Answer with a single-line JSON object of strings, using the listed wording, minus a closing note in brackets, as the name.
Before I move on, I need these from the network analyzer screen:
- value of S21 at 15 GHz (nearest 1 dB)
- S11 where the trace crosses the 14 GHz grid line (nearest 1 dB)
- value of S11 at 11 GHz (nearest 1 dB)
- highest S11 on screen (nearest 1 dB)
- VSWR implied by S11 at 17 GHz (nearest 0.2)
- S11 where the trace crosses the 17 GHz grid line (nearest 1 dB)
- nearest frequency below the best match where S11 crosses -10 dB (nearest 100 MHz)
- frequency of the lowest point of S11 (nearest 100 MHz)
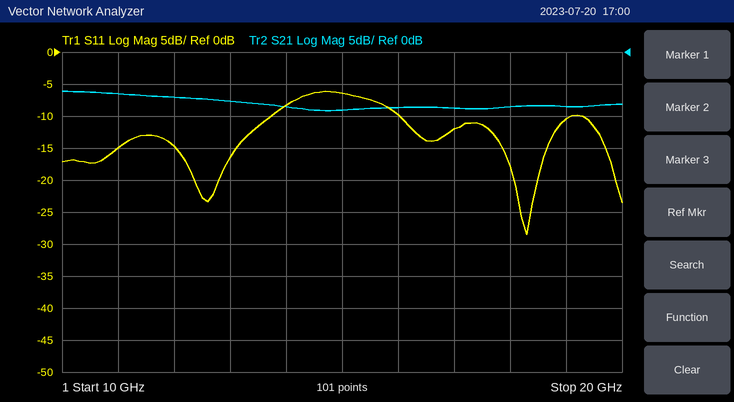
{"value of S21 at 15 GHz": "-9 dB", "S11 where the trace crosses the 14 GHz grid line": "-8 dB", "value of S11 at 11 GHz": "-15 dB", "highest S11 on screen": "-6 dB", "VSWR implied by S11 at 17 GHz": "1.6", "S11 where the trace crosses the 17 GHz grid line": "-12 dB", "nearest frequency below the best match where S11 crosses -10 dB": "16.0 GHz", "frequency of the lowest point of S11": "18.3 GHz"}
